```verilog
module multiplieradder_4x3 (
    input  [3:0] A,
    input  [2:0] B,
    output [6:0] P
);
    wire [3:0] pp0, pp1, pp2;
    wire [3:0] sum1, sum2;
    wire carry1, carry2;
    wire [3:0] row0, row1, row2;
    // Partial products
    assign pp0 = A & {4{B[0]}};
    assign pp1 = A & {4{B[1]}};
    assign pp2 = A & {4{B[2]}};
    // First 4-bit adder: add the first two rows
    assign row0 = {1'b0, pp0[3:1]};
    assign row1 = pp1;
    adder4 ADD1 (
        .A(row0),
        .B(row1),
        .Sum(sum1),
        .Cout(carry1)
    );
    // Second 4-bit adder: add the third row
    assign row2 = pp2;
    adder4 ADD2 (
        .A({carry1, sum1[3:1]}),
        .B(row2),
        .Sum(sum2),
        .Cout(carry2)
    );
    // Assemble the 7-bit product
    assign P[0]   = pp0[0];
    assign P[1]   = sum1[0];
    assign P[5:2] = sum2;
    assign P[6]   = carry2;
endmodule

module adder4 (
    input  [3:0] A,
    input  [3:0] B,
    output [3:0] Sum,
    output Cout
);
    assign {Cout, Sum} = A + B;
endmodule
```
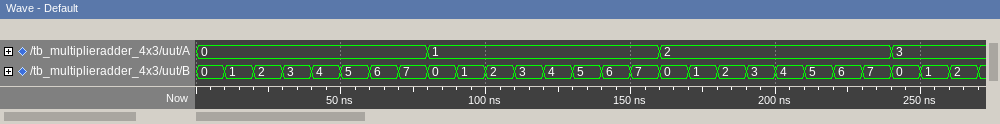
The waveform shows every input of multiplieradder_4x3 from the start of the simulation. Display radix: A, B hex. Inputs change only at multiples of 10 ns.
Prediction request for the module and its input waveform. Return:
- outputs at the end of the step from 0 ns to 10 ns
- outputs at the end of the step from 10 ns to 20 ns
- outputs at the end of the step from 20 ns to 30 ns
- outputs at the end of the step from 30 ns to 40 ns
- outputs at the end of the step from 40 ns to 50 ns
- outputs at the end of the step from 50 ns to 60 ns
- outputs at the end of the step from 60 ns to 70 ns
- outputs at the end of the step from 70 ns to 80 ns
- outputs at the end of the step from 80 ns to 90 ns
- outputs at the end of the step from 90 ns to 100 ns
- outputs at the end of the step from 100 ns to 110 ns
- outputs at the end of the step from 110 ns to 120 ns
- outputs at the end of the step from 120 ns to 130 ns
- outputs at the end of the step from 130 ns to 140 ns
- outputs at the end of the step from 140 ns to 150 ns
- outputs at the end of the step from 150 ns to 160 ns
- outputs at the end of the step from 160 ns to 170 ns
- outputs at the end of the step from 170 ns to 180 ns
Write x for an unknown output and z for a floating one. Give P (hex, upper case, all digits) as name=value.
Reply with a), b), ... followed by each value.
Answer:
a) P=00
b) P=00
c) P=00
d) P=00
e) P=00
f) P=00
g) P=00
h) P=00
i) P=00
j) P=01
k) P=02
l) P=03
m) P=04
n) P=05
o) P=06
p) P=07
q) P=00
r) P=02
